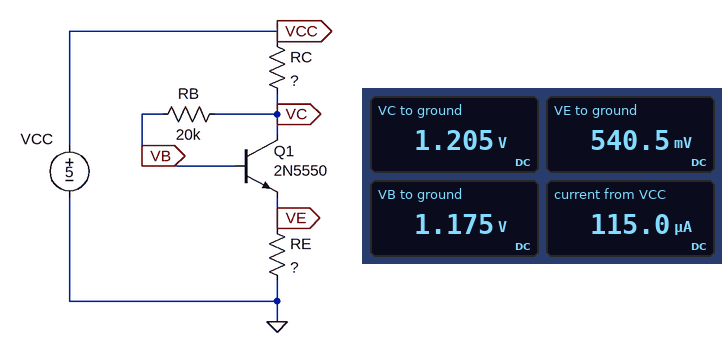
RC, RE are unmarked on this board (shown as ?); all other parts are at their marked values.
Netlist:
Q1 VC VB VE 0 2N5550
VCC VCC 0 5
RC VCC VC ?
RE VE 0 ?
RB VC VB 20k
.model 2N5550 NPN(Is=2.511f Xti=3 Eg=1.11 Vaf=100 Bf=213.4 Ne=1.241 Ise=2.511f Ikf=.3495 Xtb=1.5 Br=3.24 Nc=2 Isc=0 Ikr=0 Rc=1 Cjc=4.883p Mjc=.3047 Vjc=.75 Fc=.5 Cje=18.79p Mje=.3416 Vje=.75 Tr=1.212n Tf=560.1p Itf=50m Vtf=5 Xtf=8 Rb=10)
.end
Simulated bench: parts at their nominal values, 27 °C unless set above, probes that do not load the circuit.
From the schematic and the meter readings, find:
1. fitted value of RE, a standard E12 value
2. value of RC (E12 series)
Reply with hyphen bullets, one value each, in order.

- 4.7 kΩ
- 33 kΩ
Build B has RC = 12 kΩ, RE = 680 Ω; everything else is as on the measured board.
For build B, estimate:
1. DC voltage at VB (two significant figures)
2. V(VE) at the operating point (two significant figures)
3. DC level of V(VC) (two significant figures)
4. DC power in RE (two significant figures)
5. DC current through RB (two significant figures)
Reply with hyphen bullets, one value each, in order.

- 890 mV
- 230 mV
- 970 mV
- 77 µW
- 3.9 µA
